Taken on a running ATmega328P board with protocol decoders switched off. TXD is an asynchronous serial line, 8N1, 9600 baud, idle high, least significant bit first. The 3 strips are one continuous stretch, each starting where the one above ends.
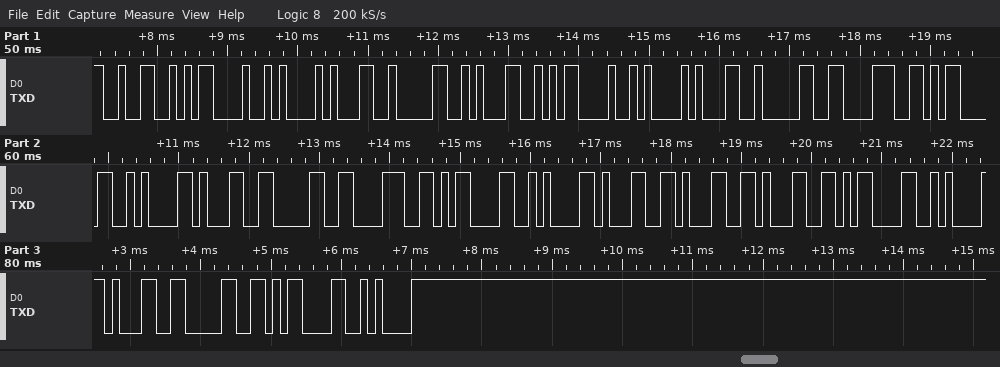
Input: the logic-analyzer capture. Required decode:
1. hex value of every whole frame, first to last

0x32 0x0D 0x0A 0x31 0x30 0x31 0x0D 0x0A 0x31 0x30 0x38 0x0D 0x0A 0x31 0x30 0x38 0x0D 0x0A 0x31 0x31 0x31 0x0D 0x0A 0x31 0x30 0x0D 0x0A
